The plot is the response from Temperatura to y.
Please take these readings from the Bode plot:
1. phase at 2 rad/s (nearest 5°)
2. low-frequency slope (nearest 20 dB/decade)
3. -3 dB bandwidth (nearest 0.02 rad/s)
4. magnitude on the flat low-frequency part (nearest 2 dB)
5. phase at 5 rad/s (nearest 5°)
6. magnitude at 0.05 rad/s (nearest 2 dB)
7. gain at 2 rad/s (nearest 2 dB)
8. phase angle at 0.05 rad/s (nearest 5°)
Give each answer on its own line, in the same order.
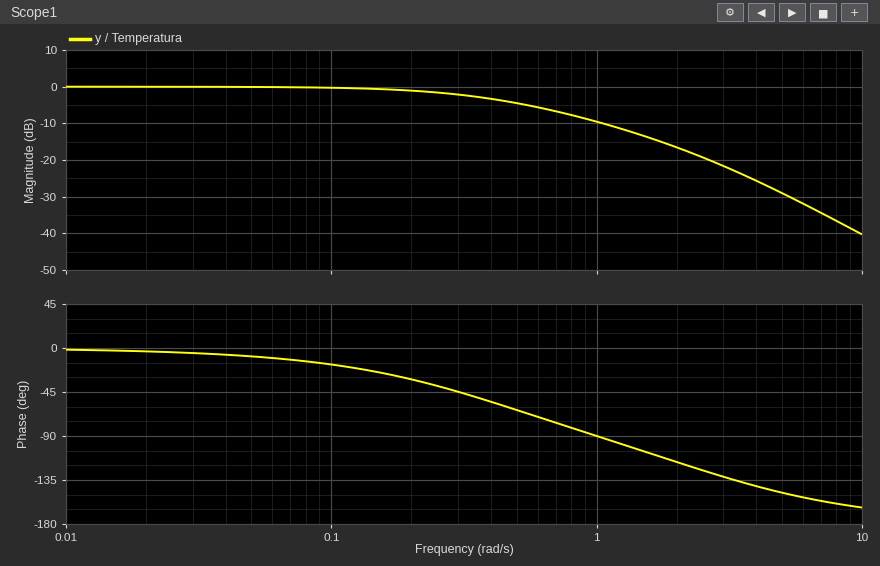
-115°
0 dB/decade
0.38 rad/s
0 dB
-150°
0 dB
-16 dB
-10°
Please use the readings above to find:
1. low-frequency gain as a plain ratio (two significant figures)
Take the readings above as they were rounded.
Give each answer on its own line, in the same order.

1.0
